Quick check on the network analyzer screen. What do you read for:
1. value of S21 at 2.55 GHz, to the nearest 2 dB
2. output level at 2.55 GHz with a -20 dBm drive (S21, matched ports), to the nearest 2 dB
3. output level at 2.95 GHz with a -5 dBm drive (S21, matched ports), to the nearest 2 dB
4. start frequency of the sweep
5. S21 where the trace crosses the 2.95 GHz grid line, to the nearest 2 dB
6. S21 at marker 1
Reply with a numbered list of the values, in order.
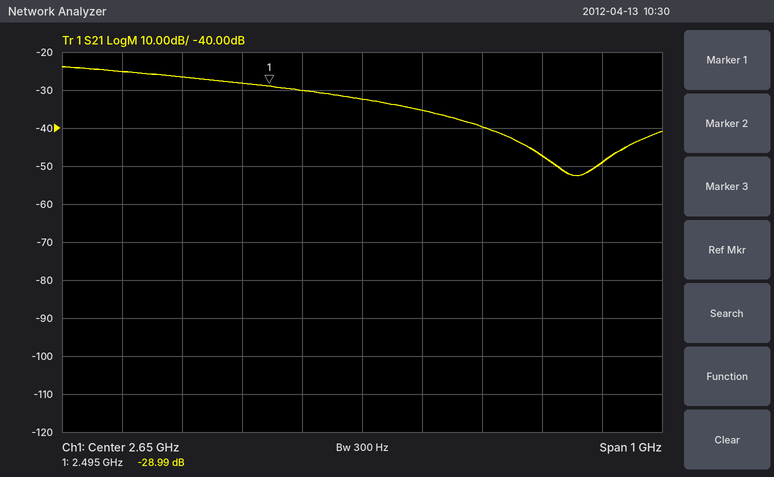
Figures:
1. -30 dB
2. -50 dBm
3. -52 dBm
4. 2.15 GHz
5. -48 dB
6. -28.99 dB
